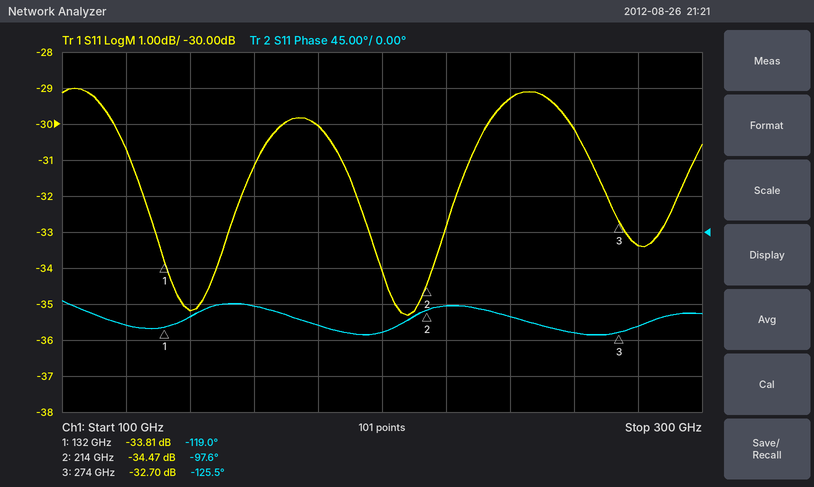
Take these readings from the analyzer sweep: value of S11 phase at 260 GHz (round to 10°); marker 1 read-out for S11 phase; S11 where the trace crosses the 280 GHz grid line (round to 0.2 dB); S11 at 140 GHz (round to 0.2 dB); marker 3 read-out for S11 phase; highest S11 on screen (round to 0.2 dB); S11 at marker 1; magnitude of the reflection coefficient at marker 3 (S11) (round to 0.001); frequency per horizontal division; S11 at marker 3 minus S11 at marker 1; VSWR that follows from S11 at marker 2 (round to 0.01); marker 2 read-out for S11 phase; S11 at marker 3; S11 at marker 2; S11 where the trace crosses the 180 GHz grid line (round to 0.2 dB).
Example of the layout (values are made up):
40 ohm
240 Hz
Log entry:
-130°
-119.0°
-33.4 dB
-35.2 dB
-125.5°
-29.0 dB
-33.81 dB
0.023
20 GHz
1.11 dB
1.04
-97.6°
-32.70 dB
-34.47 dB
-30.0 dB
